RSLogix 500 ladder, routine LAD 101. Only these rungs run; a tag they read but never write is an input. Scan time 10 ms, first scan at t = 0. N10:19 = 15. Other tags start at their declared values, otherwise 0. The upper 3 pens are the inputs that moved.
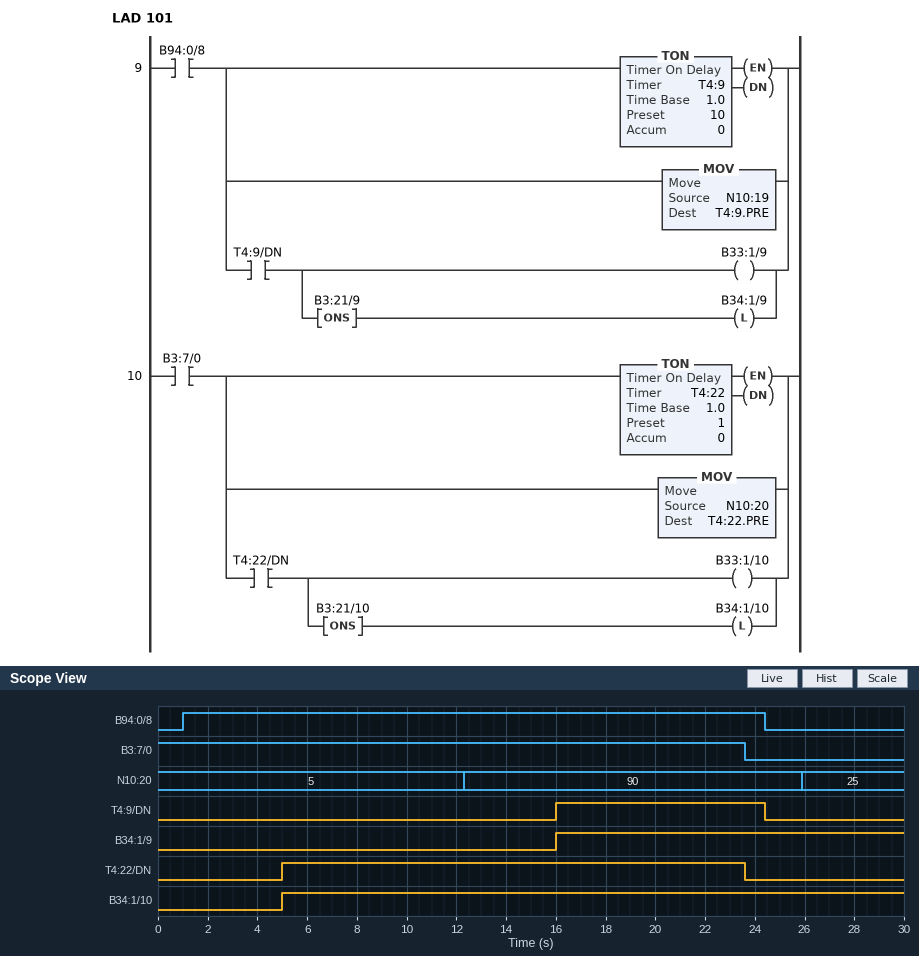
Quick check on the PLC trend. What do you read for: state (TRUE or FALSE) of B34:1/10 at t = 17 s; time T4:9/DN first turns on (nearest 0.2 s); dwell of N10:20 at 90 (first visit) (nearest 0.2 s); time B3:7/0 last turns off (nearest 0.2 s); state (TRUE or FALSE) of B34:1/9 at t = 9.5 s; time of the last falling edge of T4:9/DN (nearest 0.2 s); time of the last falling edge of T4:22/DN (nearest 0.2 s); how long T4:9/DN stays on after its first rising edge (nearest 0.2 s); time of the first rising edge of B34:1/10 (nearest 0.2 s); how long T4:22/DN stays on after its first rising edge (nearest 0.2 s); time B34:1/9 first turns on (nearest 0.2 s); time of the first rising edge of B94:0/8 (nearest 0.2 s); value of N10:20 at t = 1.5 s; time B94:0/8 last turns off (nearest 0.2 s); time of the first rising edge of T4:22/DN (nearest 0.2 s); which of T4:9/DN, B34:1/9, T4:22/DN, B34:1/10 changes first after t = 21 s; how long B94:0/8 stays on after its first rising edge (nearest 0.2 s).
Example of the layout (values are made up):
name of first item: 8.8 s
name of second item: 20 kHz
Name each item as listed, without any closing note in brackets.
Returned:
state (TRUE or FALSE) of B34:1/10 at t = 17 s: TRUE
time T4:9/DN first turns on: 16.0 s
dwell of N10:20 at 90 (first visit): 13.6 s
time B3:7/0 last turns off: 23.6 s
state (TRUE or FALSE) of B34:1/9 at t = 9.5 s: FALSE
time of the last falling edge of T4:9/DN: 24.4 s
time of the last falling edge of T4:22/DN: 23.6 s
how long T4:9/DN stays on after its first rising edge: 8.4 s
time of the first rising edge of B34:1/10: 5.0 s
how long T4:22/DN stays on after its first rising edge: 18.6 s
time B34:1/9 first turns on: 16.0 s
time of the first rising edge of B94:0/8: 1.0 s
value of N10:20 at t = 1.5 s: 5
time B94:0/8 last turns off: 24.4 s
time of the first rising edge of T4:22/DN: 5.0 s
which of T4:9/DN, B34:1/9, T4:22/DN, B34:1/10 changes first after t = 21 s: T4:22/DN
how long B94:0/8 stays on after its first rising edge: 23.4 s
